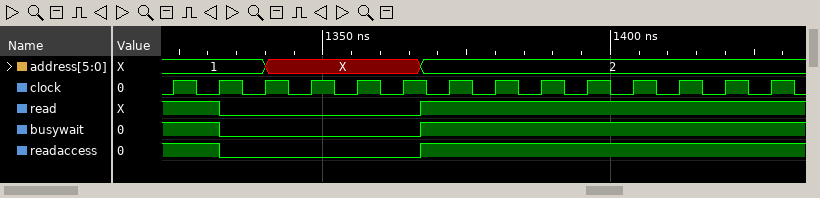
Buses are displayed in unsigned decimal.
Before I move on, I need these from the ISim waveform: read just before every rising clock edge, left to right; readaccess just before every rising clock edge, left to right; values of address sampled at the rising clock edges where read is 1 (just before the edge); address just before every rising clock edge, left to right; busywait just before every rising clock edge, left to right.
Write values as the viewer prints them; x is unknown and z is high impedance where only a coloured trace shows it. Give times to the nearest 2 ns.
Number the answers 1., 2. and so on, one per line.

1. 1 1 0 0 0 0 1 1 1 1 1 1 1 1
2. 1 1 0 0 0 0 1 1 1 1 1 1 1 1
3. 1, 1, 2, 2, 2, 2, 2, 2, 2, 2
4. 1, 1, 1, X, X, X, 2, 2, 2, 2, 2, 2, 2, 2
5. 1 1 0 0 0 0 1 1 1 1 1 1 1 1
